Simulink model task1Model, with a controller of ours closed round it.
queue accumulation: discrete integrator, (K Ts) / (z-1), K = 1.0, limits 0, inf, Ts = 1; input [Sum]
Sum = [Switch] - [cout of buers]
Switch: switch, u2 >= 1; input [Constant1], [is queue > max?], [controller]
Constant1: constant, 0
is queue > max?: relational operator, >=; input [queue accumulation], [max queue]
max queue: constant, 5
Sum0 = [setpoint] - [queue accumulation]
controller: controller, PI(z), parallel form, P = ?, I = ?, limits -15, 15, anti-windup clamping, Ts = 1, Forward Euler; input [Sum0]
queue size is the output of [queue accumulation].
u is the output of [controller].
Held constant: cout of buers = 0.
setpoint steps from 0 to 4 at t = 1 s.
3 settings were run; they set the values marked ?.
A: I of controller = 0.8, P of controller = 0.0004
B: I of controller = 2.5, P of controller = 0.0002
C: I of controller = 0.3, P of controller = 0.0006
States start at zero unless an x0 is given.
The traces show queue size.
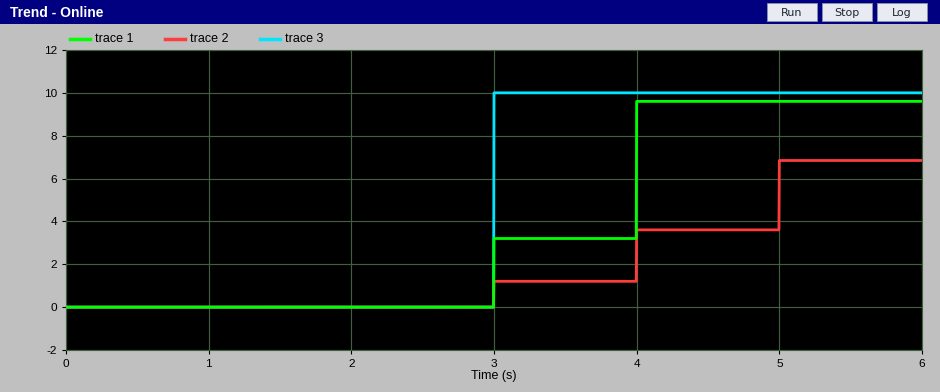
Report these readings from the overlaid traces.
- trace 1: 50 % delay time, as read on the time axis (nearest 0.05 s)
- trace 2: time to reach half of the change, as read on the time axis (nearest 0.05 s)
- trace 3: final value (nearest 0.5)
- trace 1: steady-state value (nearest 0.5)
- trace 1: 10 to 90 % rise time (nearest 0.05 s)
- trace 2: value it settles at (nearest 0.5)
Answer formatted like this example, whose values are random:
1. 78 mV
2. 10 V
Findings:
1. 4.00 s
2. 4.00 s
3. 10.0
4. 9.5
5. 1.00 s
6. 7.0
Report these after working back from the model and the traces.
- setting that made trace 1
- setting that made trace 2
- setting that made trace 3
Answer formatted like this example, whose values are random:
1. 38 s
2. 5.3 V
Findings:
1. A
2. C
3. B
